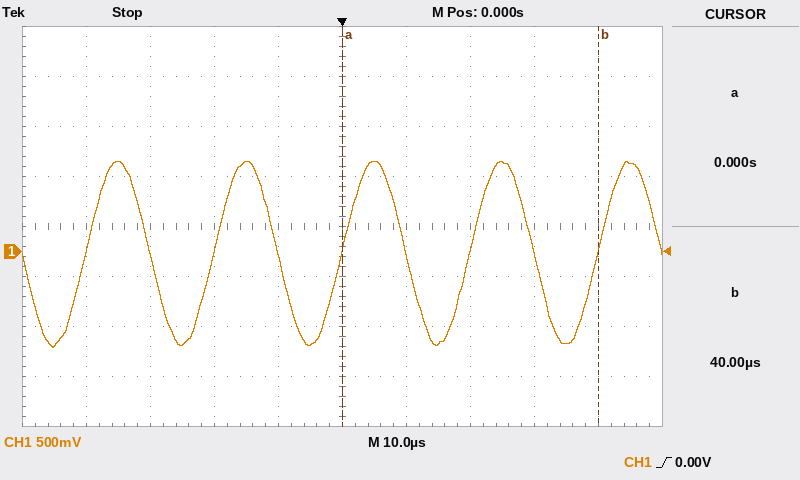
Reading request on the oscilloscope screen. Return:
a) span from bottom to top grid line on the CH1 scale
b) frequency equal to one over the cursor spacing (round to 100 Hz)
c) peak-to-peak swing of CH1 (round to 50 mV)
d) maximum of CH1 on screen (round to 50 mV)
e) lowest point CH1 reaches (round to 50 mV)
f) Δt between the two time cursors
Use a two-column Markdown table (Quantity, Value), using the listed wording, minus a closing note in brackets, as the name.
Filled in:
| Quantity | Value |
|---|---|
| span from bottom to top grid line on the CH1 scale | 4 V |
| frequency equal to one over the cursor spacing | 25.0 kHz |
| peak-to-peak swing of CH1 | 1.85 V |
| maximum of CH1 on screen | 900 mV |
| lowest point CH1 reaches | -950 mV |
| Δt between the two time cursors | 40 µs |
